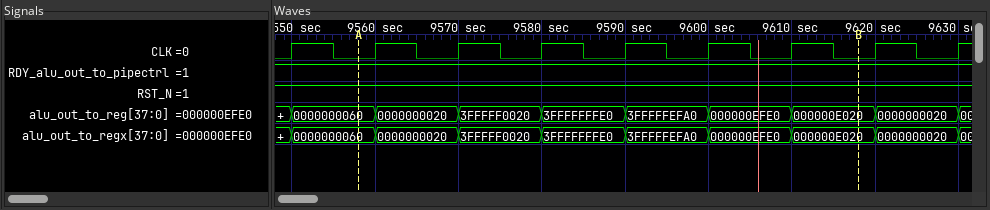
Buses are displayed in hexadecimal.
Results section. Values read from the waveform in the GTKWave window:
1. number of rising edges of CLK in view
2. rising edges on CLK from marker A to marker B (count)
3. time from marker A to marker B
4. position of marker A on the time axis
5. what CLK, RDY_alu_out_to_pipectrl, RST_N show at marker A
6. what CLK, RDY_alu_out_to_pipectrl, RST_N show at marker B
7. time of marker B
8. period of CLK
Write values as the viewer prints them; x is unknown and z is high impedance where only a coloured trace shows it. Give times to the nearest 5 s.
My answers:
9
6
60 s
9560 s
CLK=0, RDY_alu_out_to_pipectrl=1, RST_N=1
CLK=0, RDY_alu_out_to_pipectrl=1, RST_N=1
9620 s
10 s
